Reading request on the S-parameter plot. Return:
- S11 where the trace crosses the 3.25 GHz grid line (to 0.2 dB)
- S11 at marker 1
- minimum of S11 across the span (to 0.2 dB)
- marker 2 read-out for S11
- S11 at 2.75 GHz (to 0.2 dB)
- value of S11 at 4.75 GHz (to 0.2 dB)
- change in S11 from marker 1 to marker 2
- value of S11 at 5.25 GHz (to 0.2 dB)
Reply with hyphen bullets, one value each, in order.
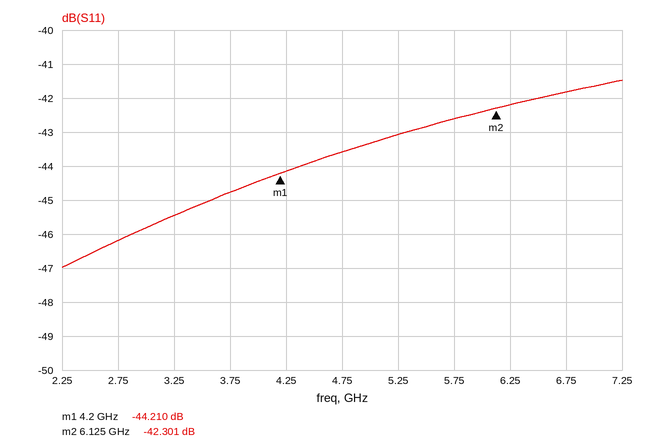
- -45.4 dB
- -44.210 dB
- -47.0 dB
- -42.301 dB
- -46.2 dB
- -43.6 dB
- 1.909 dB
- -43.0 dB
